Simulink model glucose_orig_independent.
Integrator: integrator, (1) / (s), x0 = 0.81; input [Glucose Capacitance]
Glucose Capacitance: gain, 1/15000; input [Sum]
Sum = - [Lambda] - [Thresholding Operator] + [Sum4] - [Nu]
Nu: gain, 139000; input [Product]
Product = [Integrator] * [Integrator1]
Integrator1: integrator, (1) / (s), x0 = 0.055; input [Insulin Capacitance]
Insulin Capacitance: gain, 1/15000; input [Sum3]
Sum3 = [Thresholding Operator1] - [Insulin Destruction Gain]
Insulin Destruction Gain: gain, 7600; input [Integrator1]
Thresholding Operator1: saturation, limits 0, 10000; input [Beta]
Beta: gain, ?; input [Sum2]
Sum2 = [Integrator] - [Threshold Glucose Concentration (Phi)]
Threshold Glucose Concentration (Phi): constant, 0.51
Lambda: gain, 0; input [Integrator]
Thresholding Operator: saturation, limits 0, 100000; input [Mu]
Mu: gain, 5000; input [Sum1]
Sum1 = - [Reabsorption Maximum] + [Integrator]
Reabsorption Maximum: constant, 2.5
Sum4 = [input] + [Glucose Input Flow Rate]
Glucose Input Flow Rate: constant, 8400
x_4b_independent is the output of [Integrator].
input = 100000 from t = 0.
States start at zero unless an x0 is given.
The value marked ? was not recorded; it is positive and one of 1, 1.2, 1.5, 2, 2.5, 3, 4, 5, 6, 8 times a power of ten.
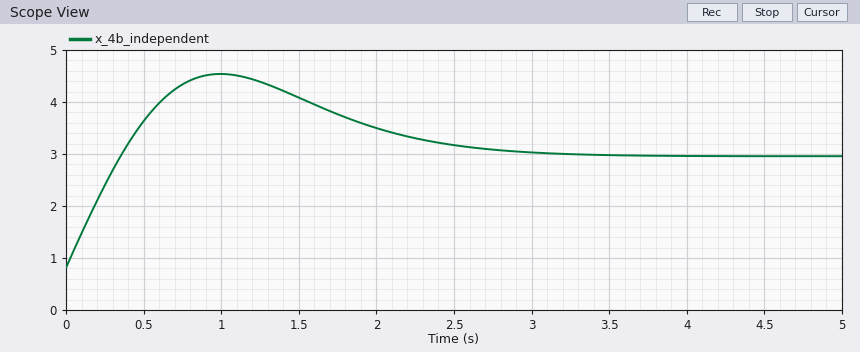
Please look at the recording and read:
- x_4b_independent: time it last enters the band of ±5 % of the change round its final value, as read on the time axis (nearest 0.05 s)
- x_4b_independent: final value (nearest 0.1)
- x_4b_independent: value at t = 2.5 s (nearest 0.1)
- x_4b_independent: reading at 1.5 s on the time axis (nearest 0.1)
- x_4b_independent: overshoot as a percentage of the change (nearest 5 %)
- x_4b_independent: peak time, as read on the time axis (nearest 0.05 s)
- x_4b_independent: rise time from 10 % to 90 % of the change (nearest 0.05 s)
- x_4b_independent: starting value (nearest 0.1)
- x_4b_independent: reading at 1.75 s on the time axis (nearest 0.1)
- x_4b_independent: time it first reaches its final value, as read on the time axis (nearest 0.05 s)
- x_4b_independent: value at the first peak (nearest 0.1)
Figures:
2.80 s
3.0
3.2
4.1
75 %
1.00 s
0.30 s
0.8
3.8
0.35 s
4.5
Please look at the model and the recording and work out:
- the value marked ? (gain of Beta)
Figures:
800
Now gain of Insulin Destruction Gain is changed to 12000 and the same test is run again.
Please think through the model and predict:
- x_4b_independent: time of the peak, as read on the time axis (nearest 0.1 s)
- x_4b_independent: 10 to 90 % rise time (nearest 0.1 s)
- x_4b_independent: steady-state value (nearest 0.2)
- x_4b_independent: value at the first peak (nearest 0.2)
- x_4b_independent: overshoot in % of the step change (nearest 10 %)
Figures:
1.1 s
0.4 s
3.6
4.8
40 %
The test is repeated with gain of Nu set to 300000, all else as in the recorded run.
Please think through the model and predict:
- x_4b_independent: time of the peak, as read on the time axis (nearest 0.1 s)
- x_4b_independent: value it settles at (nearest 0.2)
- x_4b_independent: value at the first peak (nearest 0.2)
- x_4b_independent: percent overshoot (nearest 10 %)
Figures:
0.8 s
2.2
3.2
90 %
